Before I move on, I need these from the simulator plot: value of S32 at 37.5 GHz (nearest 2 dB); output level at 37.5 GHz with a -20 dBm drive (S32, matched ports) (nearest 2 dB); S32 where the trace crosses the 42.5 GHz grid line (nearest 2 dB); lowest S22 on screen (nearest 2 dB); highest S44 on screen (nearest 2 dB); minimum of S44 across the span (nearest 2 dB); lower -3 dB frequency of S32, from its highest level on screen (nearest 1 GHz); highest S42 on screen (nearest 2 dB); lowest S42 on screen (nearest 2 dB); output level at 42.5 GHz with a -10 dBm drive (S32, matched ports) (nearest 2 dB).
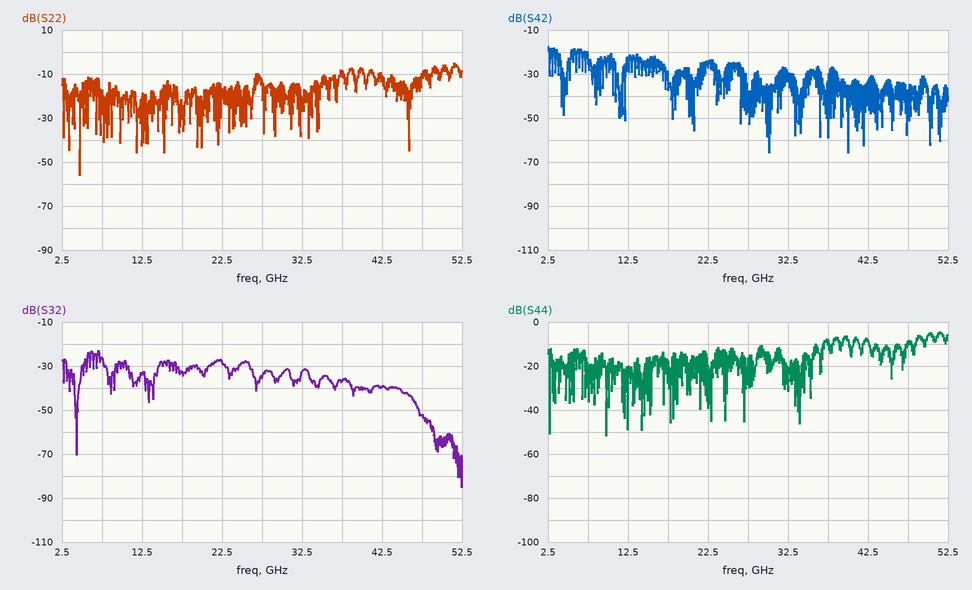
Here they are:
-36 dB
-56 dBm
-40 dB
-56 dB
-4 dB
-52 dB
7 GHz
-18 dB
-66 dB
-50 dBm
